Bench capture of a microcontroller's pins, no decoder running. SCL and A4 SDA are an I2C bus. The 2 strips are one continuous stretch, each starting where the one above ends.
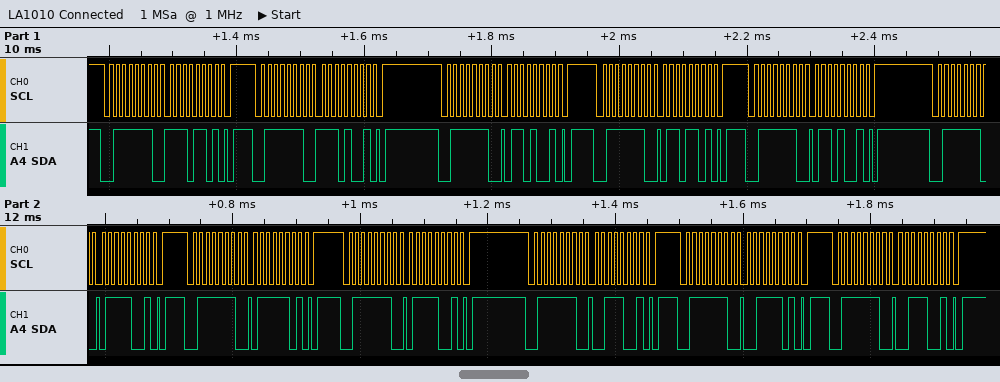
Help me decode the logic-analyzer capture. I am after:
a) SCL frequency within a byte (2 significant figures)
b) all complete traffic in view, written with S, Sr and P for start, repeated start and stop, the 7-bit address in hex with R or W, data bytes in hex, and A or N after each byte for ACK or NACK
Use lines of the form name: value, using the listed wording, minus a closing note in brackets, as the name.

SCL frequency within a byte: 100 kHz
all complete traffic in view, written with S, Sr and P for start, repeated start and stop, the 7-bit address in hex with R or W, data bytes in hex, and A or N after each byte for ACK or NACK: S 3FW A ED A P S 3FW A E9 A P S 3FW A 69 A P S 3FW A 6D A P S 3FW A 69 A P S 3FW A 79 A P S 3FW A 7D A P S 3FW A 79 A P S 3FW A 39 A P S 3FW A 3D A P S 3FW A 39 A P
